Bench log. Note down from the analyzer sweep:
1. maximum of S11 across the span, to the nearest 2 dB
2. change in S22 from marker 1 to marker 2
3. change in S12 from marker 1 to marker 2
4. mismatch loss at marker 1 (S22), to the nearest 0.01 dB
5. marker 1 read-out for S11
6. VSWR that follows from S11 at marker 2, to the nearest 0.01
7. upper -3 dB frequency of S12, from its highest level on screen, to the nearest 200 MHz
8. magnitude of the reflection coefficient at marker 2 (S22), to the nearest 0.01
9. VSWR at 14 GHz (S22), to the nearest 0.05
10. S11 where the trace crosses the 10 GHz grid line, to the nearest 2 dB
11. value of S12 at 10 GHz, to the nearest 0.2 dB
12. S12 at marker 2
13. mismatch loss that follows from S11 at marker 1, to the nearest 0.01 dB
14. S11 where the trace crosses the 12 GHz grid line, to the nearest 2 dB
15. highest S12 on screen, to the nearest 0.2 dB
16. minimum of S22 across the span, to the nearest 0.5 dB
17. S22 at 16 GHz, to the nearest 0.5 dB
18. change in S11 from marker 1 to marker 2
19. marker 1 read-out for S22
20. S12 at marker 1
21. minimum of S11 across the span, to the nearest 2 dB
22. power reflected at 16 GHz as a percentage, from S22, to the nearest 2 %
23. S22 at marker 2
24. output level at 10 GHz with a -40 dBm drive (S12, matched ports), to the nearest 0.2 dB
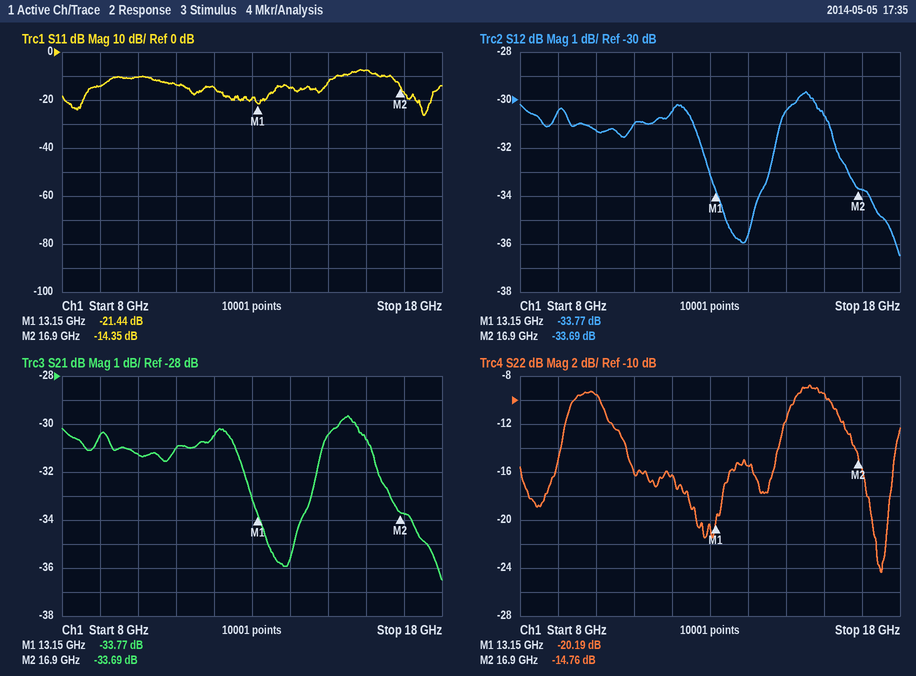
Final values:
-8 dB
5.43 dB
0.08 dB
0.04 dB
-21.44 dB
1.47
16.6 GHz
0.18
1.40
-10 dB
-31.2 dB
-33.69 dB
0.03 dB
-14 dB
-29.6 dB
-24.5 dB
-9.5 dB
7.09 dB
-20.19 dB
-33.77 dB
-26 dB
12 %
-14.76 dB
-71.2 dBm
